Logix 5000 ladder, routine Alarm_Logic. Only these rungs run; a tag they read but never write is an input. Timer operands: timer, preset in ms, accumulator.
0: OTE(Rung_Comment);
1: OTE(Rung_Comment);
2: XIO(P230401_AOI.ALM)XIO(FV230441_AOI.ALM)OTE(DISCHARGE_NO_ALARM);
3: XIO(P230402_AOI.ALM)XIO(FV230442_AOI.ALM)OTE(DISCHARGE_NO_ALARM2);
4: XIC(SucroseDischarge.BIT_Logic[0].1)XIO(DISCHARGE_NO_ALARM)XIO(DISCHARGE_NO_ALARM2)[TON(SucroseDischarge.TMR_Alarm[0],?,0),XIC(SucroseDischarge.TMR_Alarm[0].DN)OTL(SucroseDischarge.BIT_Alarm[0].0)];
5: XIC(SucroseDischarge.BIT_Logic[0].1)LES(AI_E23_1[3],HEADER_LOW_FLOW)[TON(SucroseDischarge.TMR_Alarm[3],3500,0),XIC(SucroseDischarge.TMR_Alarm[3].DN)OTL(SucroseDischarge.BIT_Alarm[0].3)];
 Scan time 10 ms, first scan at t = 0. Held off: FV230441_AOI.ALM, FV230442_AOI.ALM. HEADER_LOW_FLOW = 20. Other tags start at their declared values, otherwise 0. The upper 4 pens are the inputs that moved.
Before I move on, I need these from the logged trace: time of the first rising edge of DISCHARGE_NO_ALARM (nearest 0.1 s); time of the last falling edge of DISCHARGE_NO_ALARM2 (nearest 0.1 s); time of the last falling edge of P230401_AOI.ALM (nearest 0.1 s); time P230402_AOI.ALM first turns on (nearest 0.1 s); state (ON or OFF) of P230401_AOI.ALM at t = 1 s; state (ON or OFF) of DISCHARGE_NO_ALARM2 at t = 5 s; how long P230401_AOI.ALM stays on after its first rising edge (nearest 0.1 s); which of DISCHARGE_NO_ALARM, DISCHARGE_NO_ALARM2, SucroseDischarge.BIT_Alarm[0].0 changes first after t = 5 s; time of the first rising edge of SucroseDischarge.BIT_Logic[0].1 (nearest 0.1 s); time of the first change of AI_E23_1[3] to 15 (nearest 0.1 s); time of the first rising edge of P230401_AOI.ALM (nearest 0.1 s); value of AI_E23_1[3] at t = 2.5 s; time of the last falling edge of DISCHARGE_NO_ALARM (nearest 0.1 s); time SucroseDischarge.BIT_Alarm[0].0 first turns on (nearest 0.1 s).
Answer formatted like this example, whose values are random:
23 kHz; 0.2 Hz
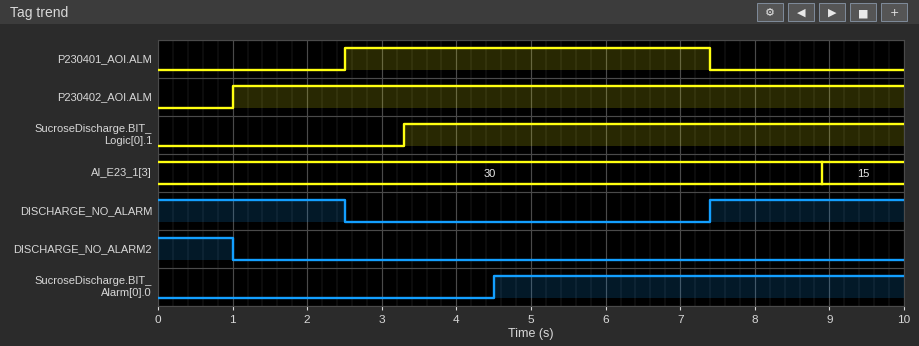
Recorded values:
7.4 s; 1.0 s; 7.4 s; 1.0 s; OFF; OFF; 4.9 s; DISCHARGE_NO_ALARM; 3.3 s; 8.9 s; 2.5 s; 30; 2.5 s; 4.5 s
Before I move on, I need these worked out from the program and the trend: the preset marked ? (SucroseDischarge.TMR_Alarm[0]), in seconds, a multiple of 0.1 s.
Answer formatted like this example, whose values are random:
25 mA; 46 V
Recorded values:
1.2 s
